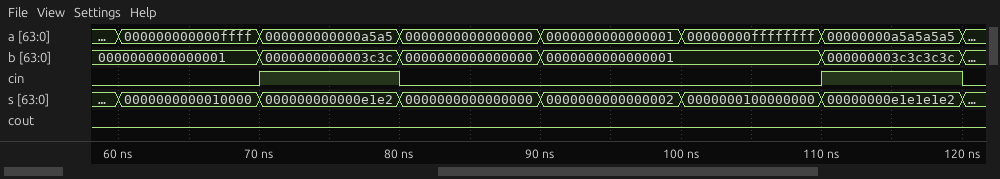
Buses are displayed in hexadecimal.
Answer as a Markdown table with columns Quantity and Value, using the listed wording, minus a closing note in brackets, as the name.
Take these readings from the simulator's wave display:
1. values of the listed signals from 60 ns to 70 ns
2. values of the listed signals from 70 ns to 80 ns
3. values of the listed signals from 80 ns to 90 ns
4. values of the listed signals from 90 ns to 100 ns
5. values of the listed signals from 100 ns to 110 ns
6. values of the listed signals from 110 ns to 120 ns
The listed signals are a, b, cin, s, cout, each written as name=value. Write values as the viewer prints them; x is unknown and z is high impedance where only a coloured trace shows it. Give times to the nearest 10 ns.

| Quantity | Value |
|---|---|
| values of the listed signals from 60 ns to 70 ns | a=000000000000ffff, b=0000000000000001, cin=0, s=0000000000010000, cout=0 |
| values of the listed signals from 70 ns to 80 ns | a=000000000000a5a5, b=0000000000003c3c, cin=1, s=000000000000e1e2, cout=0 |
| values of the listed signals from 80 ns to 90 ns | a=0000000000000000, b=0000000000000000, cin=0, s=0000000000000000, cout=0 |
| values of the listed signals from 90 ns to 100 ns | a=0000000000000001, b=0000000000000001, cin=0, s=0000000000000002, cout=0 |
| values of the listed signals from 100 ns to 110 ns | a=00000000ffffffff, b=0000000000000001, cin=0, s=0000000100000000, cout=0 |
| values of the listed signals from 110 ns to 120 ns | a=00000000a5a5a5a5, b=000000003c3c3c3c, cin=1, s=00000000e1e1e1e2, cout=0 |
